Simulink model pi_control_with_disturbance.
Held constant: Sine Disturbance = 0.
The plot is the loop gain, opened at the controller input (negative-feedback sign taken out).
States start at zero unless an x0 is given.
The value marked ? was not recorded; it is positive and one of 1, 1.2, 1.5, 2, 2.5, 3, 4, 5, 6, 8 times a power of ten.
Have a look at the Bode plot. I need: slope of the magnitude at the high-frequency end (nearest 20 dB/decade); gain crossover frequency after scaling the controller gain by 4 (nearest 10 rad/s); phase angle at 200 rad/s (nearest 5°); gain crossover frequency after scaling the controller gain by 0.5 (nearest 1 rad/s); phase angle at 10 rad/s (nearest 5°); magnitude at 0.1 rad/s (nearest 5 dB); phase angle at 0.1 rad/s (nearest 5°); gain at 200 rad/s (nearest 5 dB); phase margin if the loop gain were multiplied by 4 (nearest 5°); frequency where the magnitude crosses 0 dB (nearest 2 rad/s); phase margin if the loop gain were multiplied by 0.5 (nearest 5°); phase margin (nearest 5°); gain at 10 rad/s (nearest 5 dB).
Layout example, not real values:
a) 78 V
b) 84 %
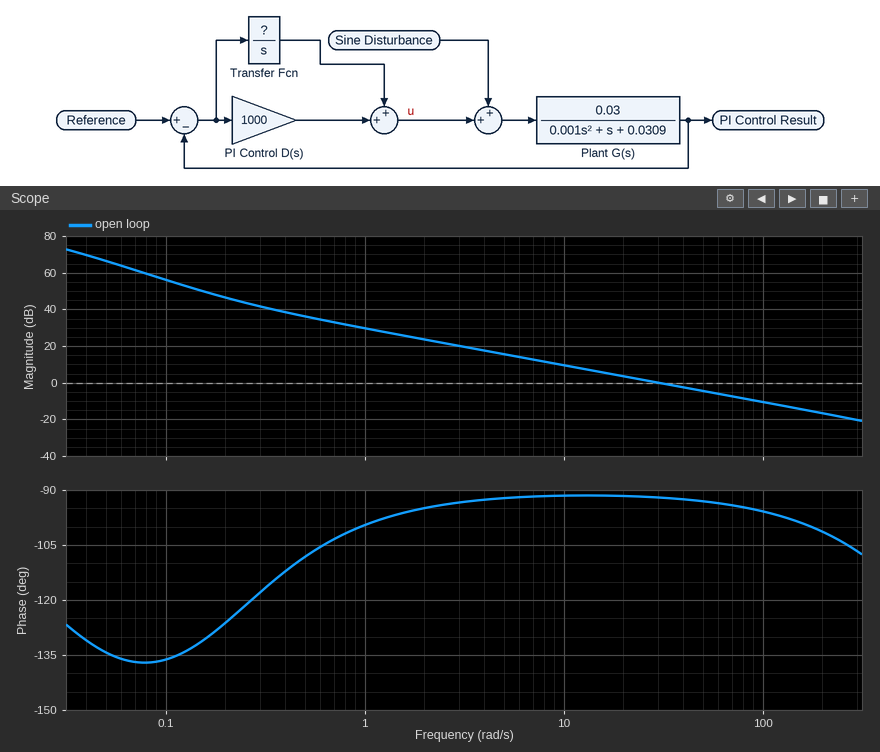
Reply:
a) -20 dB/decade
b) 120 rad/s
c) -100°
d) 15 rad/s
e) -90°
f) 55 dB
g) -135°
h) -15 dB
i) 85°
j) 30 rad/s
k) 90°
l) 90°
m) 10 dB
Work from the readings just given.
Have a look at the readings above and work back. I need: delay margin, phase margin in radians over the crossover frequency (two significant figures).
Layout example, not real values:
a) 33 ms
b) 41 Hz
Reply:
a) 0.052 s
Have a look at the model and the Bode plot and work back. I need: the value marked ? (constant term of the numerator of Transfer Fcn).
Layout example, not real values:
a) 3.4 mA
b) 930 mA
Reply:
a) 200
